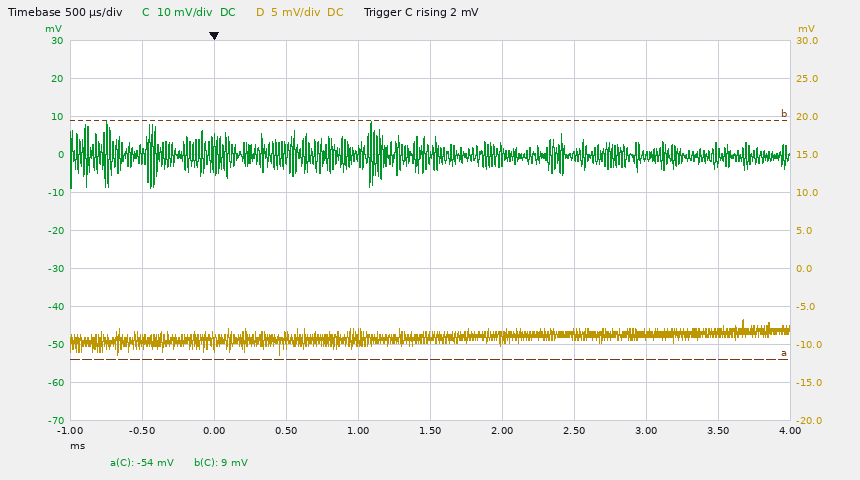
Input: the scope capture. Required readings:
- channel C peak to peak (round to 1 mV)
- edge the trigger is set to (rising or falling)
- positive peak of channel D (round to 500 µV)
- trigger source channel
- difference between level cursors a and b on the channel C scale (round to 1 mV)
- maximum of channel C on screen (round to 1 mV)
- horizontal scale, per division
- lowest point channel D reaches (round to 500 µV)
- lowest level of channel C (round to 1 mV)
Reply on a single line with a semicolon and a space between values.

18 mV; rising; -6.5 mV; channel C; 63 mV; 9 mV; 500 µs; -11.5 mV; -9 mV
